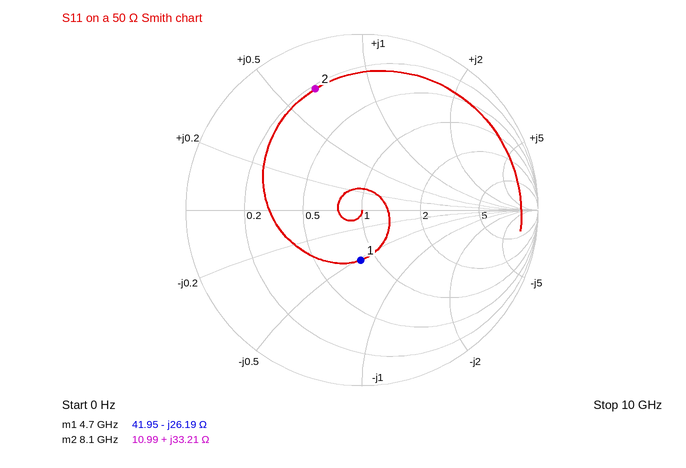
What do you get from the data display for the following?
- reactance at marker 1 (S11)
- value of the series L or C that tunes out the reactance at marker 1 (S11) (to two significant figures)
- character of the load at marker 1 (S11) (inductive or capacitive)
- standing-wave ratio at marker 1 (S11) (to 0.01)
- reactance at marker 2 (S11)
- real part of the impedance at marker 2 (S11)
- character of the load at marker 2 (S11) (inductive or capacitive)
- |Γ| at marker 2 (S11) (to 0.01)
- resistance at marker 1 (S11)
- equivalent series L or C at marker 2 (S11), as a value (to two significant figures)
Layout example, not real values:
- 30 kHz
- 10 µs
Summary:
- -26.19 Ω
- 890 pH
- capacitive
- 1.80
- +33.21 Ω
- 10.99 Ω
- inductive
- 0.74
- 41.95 Ω
- 650 pH
